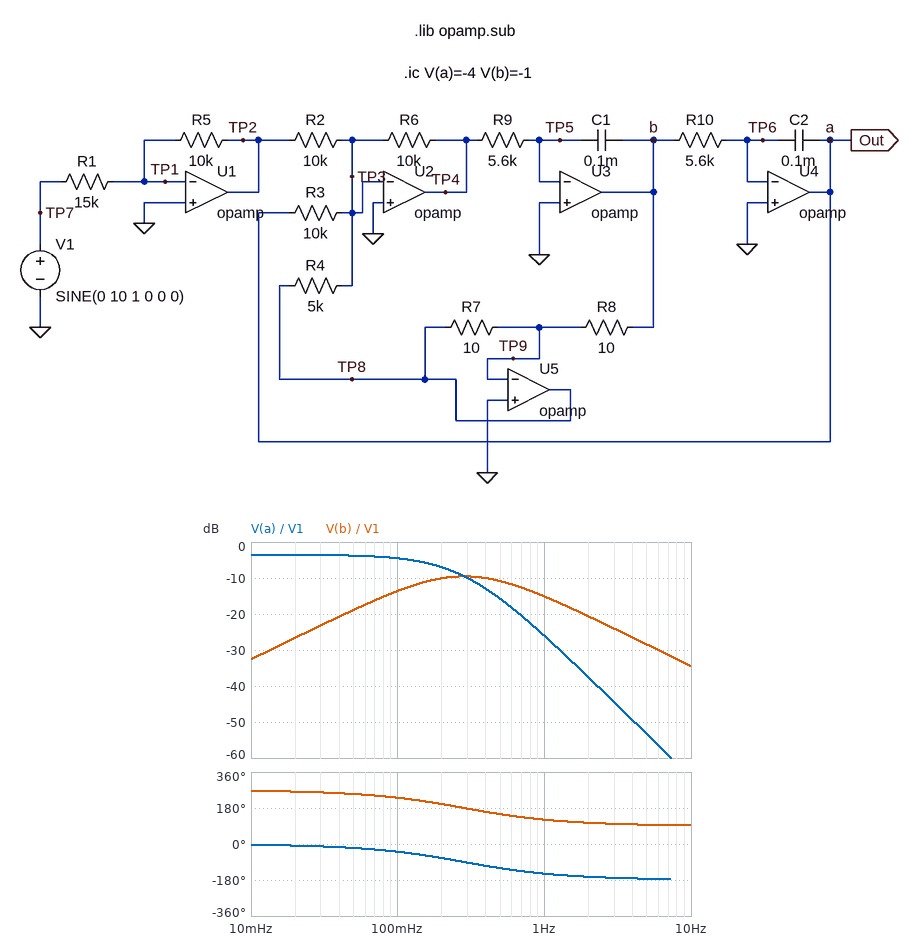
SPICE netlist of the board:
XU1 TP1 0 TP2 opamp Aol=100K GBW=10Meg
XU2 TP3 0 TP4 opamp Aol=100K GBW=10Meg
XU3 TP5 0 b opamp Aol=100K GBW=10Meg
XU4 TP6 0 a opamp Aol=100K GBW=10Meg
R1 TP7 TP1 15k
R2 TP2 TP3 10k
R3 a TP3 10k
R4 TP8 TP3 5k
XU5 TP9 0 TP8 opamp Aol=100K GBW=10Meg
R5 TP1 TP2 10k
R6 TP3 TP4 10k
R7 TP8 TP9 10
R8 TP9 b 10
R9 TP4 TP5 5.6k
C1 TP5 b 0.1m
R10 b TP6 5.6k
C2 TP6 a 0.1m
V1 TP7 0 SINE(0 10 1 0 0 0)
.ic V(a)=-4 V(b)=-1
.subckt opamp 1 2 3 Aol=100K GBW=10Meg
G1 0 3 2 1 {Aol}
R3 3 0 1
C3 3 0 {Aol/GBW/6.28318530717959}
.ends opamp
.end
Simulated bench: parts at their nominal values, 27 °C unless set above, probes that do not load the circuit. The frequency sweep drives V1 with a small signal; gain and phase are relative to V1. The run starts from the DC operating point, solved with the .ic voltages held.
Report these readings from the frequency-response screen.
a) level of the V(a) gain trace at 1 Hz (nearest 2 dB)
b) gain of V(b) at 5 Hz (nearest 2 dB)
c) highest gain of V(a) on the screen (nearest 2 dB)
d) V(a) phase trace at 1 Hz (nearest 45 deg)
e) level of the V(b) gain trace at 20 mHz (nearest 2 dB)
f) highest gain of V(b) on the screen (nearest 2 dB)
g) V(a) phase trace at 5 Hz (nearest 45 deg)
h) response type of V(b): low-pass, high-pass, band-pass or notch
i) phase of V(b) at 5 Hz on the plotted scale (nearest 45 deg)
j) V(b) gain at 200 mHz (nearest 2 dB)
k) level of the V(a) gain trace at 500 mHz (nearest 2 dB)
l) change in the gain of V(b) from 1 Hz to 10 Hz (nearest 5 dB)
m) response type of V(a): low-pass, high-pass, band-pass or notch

-26 dB
-28 dB
-4 dB
-135 deg
-26 dB
-10 dB
-180 deg
band-pass
90 deg
-10 dB
-16 dB
-20 dB
low-pass
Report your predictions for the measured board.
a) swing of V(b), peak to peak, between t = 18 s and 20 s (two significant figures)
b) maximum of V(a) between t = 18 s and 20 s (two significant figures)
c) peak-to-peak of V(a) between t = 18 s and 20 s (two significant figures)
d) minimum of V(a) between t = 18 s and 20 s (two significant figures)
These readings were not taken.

3.5 V
500 mV
1.0 V
-500 mV
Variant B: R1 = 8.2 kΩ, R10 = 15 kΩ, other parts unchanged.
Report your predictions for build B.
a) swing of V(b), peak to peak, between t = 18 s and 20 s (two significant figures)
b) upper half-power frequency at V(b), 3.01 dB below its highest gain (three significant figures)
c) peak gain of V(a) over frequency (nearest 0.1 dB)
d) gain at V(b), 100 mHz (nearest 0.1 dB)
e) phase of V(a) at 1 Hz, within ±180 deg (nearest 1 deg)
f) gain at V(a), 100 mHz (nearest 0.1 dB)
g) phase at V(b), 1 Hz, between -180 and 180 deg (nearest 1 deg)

6.2 V
617 mHz
1.7 dB
-4.8 dB
-150 deg
-4.3 dB
120 deg
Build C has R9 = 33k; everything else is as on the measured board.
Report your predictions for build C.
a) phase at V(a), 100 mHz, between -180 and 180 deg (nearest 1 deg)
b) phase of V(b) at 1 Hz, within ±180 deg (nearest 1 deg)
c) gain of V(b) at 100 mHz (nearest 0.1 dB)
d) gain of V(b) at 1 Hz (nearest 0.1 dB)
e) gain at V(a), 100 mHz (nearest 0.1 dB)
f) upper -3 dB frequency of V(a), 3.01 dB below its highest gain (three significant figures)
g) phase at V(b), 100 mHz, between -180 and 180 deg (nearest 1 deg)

-69 deg
96 deg
-10.1 dB
-29.8 dB
-1.1 dB
139 mHz
-159 deg
